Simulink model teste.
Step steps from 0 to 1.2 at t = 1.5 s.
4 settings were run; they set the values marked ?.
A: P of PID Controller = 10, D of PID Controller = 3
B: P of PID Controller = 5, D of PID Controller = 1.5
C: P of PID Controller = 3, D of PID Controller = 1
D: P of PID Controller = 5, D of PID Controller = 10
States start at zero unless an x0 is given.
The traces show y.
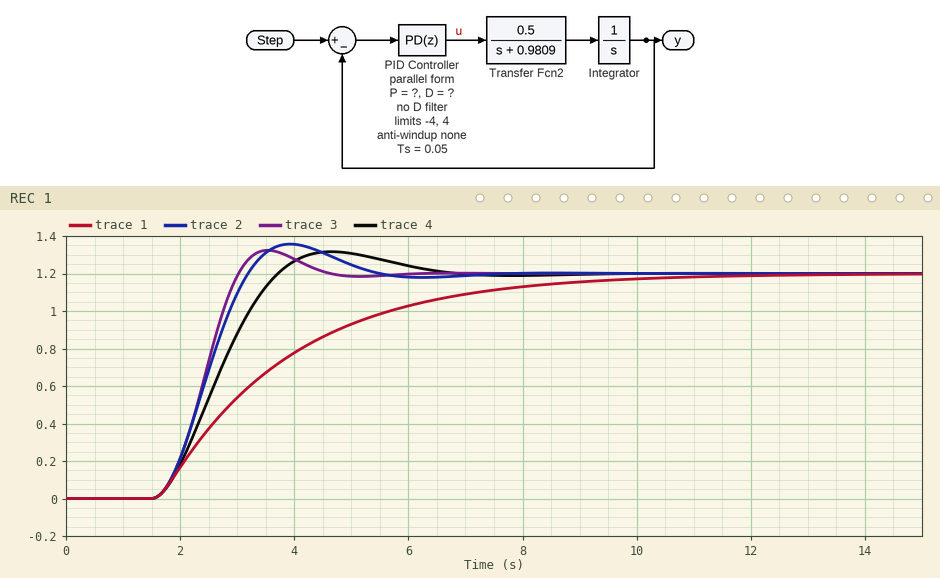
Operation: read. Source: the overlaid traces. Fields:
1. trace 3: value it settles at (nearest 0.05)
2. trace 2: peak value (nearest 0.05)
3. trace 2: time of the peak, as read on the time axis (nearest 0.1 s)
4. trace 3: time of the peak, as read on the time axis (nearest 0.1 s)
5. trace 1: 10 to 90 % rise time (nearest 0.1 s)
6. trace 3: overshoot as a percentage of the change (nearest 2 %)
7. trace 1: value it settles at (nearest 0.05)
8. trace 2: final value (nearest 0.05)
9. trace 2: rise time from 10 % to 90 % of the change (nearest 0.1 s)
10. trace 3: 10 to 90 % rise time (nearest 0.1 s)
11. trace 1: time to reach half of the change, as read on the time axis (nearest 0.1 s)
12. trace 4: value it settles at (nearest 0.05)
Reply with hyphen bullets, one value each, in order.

- 1.20
- 1.35
- 3.9 s
- 3.5 s
- 4.9 s
- 10 %
- 1.20
- 1.20
- 1.1 s
- 1.0 s
- 3.2 s
- 1.20
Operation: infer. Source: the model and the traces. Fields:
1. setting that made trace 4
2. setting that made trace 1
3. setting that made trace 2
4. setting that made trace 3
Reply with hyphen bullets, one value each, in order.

- C
- D
- B
- A
